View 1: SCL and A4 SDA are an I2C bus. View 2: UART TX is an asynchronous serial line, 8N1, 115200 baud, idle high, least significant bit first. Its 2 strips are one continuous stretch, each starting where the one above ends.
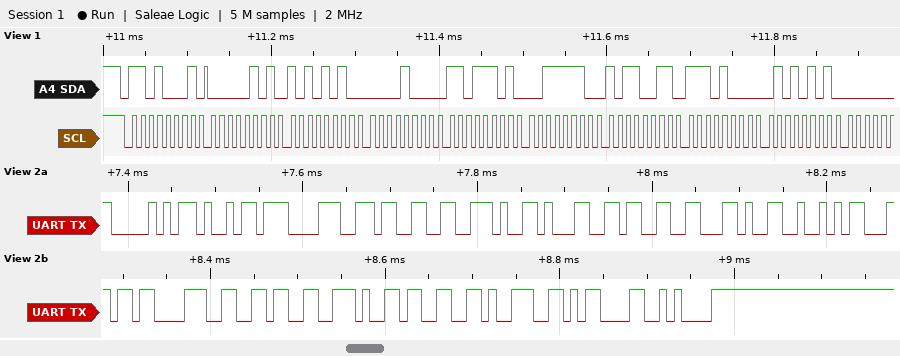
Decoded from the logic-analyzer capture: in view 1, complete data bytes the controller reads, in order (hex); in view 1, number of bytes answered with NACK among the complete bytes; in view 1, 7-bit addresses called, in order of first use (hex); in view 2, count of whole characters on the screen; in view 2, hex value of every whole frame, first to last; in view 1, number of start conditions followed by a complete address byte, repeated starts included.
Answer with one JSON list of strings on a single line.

["05 AA 08 DD 3E B3 E8 55", "0", "0x68", "17", "0x50 0x69 0x38 0x33 0x2E 0x31 0x33 0x2C 0x52 0x6C 0x38 0x36 0x2E 0x33 0x39 0x0D 0x0A", "1"]
